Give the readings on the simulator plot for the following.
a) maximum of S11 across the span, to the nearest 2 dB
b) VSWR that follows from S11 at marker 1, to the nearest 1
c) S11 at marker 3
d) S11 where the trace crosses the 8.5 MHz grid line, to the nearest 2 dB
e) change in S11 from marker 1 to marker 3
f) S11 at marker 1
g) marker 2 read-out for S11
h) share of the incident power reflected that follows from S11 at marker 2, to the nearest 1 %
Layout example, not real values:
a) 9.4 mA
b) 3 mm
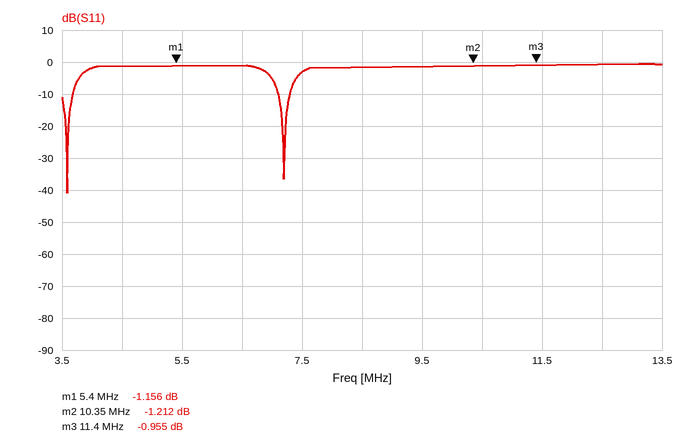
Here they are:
a) 0 dB
b) 15
c) -0.955 dB
d) -2 dB
e) 0.201 dB
f) -1.156 dB
g) -1.212 dB
h) 76 %
